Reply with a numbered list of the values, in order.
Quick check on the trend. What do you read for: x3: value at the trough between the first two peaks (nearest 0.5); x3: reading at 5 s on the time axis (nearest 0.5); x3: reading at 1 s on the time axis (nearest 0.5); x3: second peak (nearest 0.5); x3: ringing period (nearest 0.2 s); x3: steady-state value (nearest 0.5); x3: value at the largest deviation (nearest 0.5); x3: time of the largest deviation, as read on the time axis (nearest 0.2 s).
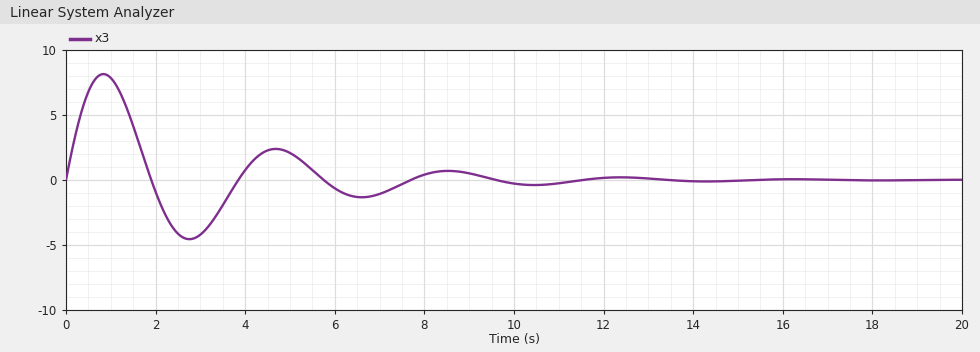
1. -4.5
2. 2.0
3. 8.0
4. 2.5
5. 3.8 s
6. 0.0
7. 8.0
8. 0.8 s
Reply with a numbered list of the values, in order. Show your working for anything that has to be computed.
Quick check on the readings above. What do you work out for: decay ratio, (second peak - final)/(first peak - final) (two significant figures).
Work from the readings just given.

1. (2.5 - 0) / (8 - 0) = 0.31
